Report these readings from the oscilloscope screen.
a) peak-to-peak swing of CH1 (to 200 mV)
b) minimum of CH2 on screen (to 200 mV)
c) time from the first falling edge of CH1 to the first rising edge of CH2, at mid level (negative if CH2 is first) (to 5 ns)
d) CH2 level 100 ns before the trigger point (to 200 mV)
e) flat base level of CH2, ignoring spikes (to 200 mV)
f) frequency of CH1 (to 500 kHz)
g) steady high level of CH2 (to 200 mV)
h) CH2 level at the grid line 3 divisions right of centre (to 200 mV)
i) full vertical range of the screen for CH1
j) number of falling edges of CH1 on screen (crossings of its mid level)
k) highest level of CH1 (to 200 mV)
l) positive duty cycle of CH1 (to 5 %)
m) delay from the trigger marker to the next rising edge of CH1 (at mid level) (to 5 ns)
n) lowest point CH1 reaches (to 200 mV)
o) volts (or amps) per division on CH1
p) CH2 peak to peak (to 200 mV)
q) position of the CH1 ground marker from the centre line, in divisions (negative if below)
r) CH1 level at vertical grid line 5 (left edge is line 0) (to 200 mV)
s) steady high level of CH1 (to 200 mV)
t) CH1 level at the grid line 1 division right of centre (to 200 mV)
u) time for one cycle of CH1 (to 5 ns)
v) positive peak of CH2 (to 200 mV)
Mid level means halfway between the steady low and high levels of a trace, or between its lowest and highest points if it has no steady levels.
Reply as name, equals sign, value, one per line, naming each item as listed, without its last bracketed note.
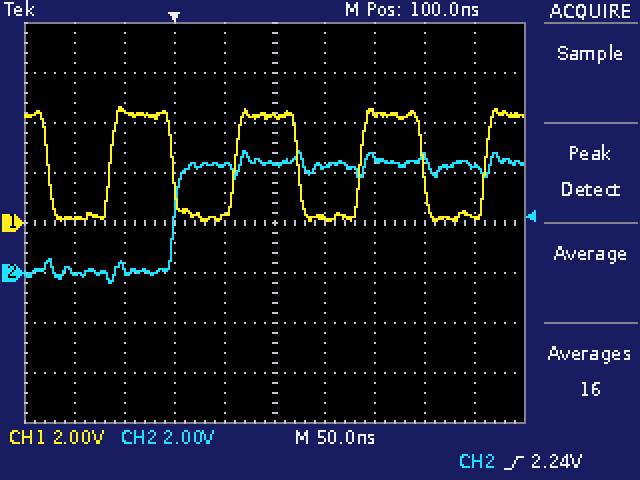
peak-to-peak swing of CH1 = 4.6 V
minimum of CH2 on screen = -400 mV
time from the first falling edge of CH1 to the first rising edge of CH2, at mid level (negative if CH2 is first) = +125 ns
CH2 level 100 ns before the trigger point = 0.0 V
flat base level of CH2, ignoring spikes = 0.0 V
frequency of CH1 = 8.0 MHz
steady high level of CH2 = 4.4 V
CH2 level at the grid line 3 divisions right of centre = 4.6 V
full vertical range of the screen for CH1 = 16 V
number of falling edges of CH1 on screen = 4
highest level of CH1 = 4.6 V
positive duty cycle of CH1 = 50 %
delay from the trigger marker to the next rising edge of CH1 (at mid level) = 60 ns
lowest point CH1 reaches = 0.0 V
volts (or amps) per division on CH1 = 2 V
CH2 peak to peak = 5.2 V
position of the CH1 ground marker from the centre line, in divisions = 0.0 div
CH1 level at vertical grid line 5 (left edge is line 0) = 4.2 V
steady high level of CH1 = 4.4 V
CH1 level at the grid line 1 division right of centre = 200 mV
time for one cycle of CH1 = 125 ns
positive peak of CH2 = 4.8 V
